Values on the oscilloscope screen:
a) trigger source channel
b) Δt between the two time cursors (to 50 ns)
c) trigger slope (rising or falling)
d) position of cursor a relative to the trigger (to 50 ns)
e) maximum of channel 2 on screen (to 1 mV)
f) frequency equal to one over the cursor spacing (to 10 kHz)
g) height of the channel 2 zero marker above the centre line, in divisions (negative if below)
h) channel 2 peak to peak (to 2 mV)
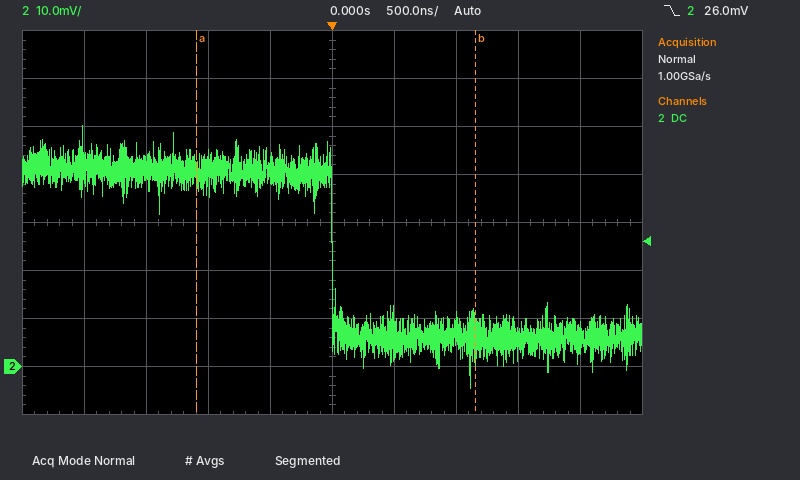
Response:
channel 2
2.25 µs
falling
-1.10 µs
50 mV
440 kHz
-3.0 div
54 mV
